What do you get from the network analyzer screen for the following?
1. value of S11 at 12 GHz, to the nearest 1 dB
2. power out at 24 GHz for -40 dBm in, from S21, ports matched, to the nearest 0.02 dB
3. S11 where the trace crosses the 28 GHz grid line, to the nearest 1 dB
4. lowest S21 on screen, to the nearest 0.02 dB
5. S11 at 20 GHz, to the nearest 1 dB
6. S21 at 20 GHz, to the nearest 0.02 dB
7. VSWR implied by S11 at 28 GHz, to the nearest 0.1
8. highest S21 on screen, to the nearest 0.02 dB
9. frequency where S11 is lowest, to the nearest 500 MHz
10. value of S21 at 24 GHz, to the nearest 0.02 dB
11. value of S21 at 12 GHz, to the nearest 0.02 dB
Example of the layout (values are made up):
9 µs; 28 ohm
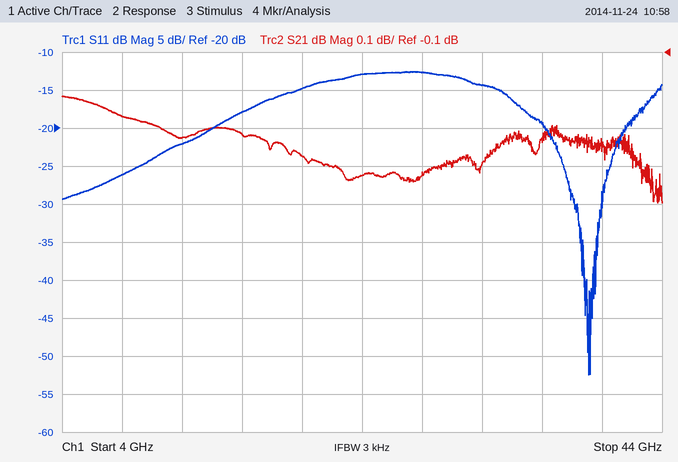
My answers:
-22 dB; -40.42 dBm; -13 dB; -0.50 dB; -15 dB; -0.38 dB; 1.6; -0.22 dB; 39.0 GHz; -0.42 dB; -0.32 dB
